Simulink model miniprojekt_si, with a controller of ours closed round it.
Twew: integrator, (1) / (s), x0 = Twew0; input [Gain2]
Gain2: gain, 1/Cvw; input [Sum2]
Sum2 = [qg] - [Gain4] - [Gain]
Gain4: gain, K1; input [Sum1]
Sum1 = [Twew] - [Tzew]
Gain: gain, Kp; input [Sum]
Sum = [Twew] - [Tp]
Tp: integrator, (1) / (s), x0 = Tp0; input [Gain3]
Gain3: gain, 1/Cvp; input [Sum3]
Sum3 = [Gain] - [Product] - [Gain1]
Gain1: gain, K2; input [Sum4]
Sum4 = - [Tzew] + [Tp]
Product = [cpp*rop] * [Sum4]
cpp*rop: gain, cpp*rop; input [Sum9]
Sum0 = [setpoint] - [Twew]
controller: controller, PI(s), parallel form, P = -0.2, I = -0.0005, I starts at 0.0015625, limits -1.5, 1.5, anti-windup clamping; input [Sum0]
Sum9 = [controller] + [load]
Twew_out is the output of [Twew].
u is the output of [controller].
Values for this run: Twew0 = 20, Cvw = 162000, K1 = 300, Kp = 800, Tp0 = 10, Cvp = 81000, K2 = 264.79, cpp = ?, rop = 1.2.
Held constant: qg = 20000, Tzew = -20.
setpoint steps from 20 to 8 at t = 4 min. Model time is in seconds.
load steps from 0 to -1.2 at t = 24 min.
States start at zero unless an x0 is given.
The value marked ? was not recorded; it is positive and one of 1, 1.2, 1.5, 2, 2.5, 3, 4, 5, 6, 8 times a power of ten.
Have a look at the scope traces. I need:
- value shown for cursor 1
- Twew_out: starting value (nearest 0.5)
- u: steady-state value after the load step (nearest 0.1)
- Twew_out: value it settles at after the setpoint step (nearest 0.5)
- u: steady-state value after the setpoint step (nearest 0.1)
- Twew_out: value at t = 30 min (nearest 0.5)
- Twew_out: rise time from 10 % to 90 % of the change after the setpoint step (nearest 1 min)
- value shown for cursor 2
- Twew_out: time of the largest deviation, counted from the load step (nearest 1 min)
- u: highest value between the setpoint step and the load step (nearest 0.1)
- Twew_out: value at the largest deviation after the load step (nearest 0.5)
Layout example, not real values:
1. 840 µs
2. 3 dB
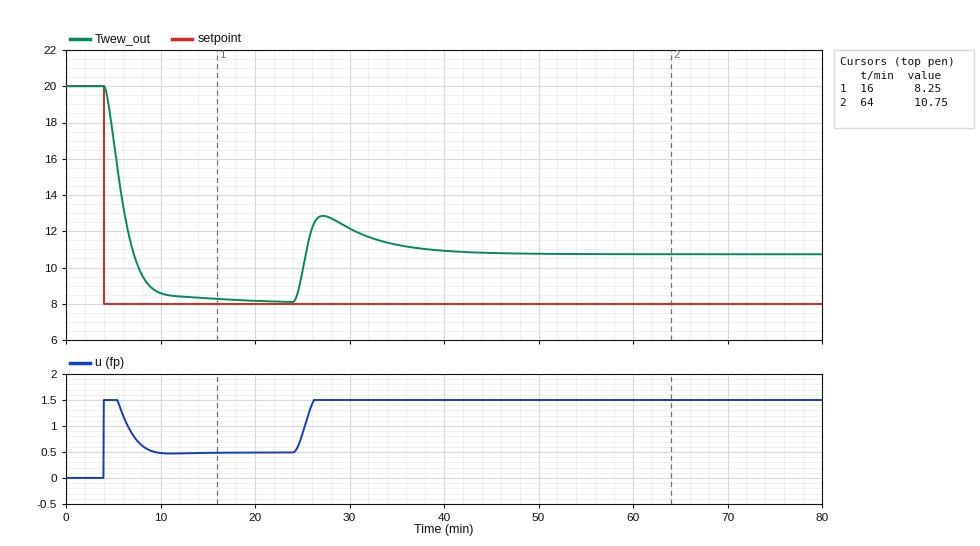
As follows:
1. 8.25
2. 20.0
3. 1.5
4. 8.0
5. 0.5
6. 12.0
7. 4 min
8. 10.75
9. 3 min
10. 1.5
11. 13.0
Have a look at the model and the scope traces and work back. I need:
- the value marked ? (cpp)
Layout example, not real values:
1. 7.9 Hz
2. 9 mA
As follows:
1. 1000
